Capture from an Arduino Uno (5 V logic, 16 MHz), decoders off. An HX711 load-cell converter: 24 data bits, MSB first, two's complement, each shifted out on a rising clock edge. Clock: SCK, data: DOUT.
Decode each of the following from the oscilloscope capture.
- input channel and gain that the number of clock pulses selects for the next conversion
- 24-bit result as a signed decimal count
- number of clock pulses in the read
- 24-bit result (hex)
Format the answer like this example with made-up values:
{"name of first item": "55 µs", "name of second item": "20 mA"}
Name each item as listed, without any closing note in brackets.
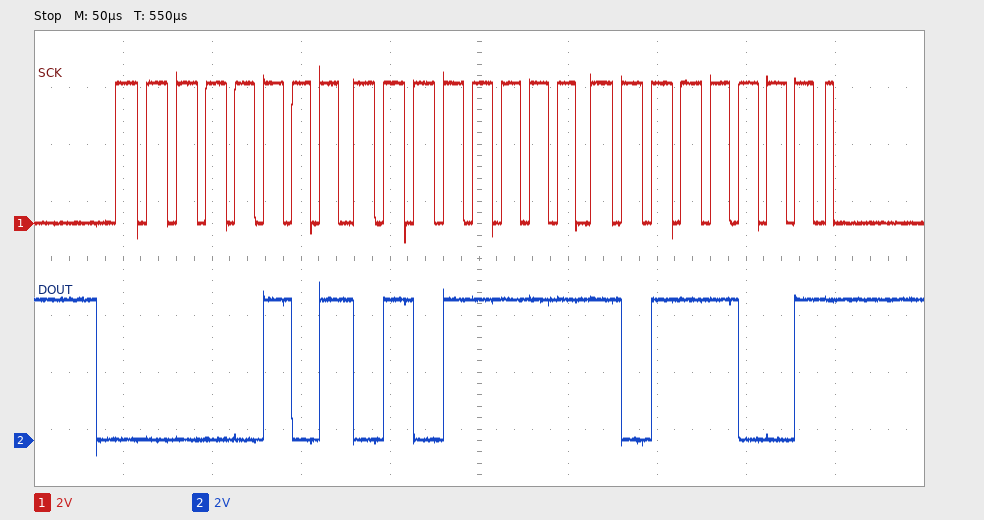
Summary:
{"input channel and gain that the number of clock pulses selects for the next conversion": "channel A, gain 128", "24-bit result as a signed decimal count": "352185", "number of clock pulses in the read": "25", "24-bit result": "0x055FB9"}
